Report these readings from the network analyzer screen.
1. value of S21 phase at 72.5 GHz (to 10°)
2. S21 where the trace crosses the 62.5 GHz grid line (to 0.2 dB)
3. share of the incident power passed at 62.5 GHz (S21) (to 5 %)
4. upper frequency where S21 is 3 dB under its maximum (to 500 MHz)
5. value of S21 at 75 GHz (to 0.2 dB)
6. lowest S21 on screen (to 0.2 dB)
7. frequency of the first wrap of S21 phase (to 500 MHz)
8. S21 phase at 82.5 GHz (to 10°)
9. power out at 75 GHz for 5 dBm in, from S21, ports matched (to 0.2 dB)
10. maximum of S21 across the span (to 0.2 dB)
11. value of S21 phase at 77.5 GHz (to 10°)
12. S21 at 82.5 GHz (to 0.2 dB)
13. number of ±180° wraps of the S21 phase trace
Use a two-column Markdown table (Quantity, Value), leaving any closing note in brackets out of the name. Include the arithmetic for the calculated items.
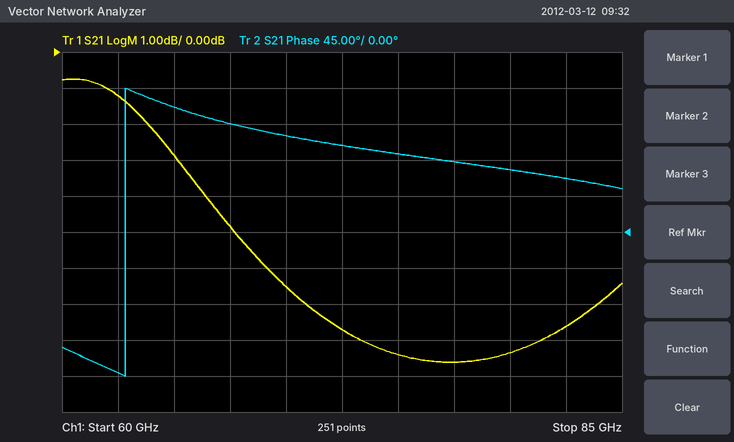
| Quantity | Value |
|---|---|
| value of S21 phase at 72.5 GHz | 110° |
| S21 where the trace crosses the 62.5 GHz grid line | -1.2 dB |
| share of the incident power passed at 62.5 GHz (S21) | 10^(-1.2/10) ≈ 75.9 %, so 75 % to the nearest 5 % |
| upper frequency where S21 is 3 dB under its maximum | 66.0 GHz |
| value of S21 at 75 GHz | -8.4 dB |
| lowest S21 on screen | -8.6 dB |
| frequency of the first wrap of S21 phase | 63.0 GHz |
| S21 phase at 82.5 GHz | 70° |
| power out at 75 GHz for 5 dBm in, from S21, ports matched | 5 dBm + (-8.4 dB) = -3.4 dBm |
| maximum of S21 across the span | -0.8 dB |
| value of S21 phase at 77.5 GHz | 90° |
| S21 at 82.5 GHz | -7.6 dB |
| number of ±180° wraps of the S21 phase trace | 1 |
